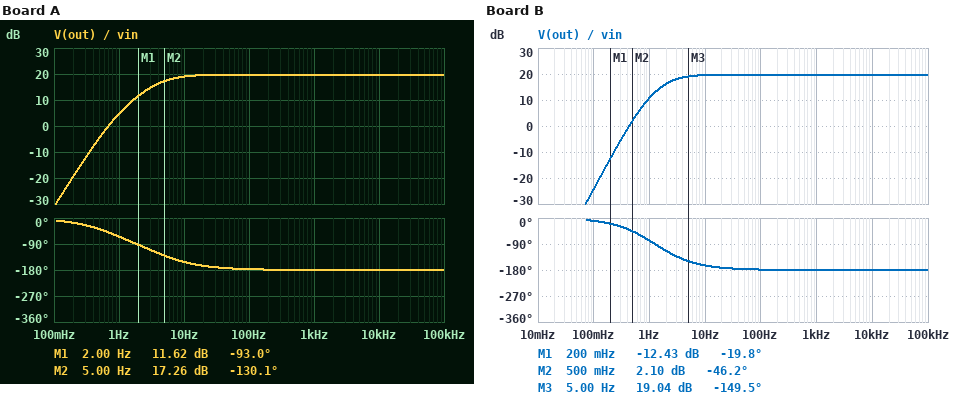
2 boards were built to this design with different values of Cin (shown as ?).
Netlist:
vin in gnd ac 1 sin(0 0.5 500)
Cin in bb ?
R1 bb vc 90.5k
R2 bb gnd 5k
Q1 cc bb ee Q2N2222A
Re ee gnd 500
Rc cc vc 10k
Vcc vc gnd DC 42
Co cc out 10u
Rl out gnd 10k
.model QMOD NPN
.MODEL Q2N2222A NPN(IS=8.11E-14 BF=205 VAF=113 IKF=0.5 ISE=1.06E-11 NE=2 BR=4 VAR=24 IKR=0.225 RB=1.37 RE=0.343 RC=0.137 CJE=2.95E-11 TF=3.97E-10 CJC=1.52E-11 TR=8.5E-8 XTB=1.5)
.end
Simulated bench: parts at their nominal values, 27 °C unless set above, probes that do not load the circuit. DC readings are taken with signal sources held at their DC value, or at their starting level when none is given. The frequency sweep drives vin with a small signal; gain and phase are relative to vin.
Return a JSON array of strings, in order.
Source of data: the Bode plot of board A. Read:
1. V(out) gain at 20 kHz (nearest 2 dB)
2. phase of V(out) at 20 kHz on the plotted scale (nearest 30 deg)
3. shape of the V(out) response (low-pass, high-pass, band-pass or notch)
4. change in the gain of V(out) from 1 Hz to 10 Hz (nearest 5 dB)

["20 dB", "-180 deg", "high-pass", "15 dB"]
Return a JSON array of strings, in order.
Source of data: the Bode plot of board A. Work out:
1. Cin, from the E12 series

["8.2 µF"]
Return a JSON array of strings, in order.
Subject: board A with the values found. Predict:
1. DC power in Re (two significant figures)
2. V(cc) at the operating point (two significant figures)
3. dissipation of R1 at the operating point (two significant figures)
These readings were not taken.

["4.5 mW", "12 V", "18 mW"]
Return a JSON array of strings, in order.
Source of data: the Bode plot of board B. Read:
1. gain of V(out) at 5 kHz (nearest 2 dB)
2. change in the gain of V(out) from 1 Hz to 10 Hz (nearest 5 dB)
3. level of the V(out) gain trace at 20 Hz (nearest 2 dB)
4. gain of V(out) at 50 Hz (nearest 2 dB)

["20 dB", "10 dB", "20 dB", "20 dB"]
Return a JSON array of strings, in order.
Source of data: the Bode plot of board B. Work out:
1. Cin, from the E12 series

["18 µF"]
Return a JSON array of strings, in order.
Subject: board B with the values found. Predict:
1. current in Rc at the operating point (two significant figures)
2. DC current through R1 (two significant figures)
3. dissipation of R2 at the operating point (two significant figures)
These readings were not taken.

["3.0 mA", "440 µA", "900 µW"]
